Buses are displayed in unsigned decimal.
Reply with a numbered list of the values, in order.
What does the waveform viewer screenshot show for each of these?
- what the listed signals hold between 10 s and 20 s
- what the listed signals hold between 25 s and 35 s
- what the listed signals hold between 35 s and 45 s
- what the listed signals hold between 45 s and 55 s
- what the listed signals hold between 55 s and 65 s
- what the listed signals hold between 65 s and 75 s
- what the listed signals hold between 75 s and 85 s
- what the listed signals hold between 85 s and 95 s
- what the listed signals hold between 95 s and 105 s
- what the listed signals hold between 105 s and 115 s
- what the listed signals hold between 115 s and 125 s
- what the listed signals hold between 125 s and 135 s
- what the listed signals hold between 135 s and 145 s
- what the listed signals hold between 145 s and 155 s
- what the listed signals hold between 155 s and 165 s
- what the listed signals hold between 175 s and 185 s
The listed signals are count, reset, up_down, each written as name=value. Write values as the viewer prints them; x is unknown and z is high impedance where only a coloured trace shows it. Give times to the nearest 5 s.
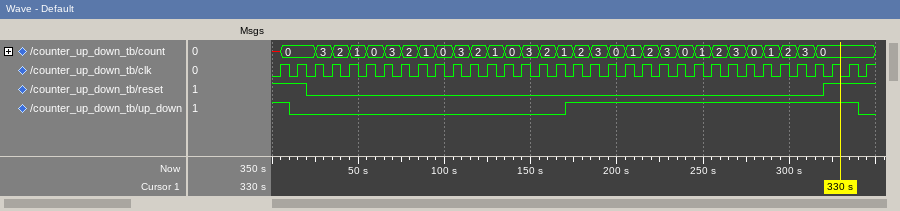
1. count=0, reset=1, up_down=0
2. count=3, reset=0, up_down=0
3. count=2, reset=0, up_down=0
4. count=1, reset=0, up_down=0
5. count=0, reset=0, up_down=0
6. count=3, reset=0, up_down=0
7. count=2, reset=0, up_down=0
8. count=1, reset=0, up_down=0
9. count=0, reset=0, up_down=0
10. count=3, reset=0, up_down=0
11. count=2, reset=0, up_down=0
12. count=1, reset=0, up_down=0
13. count=0, reset=0, up_down=0
14. count=3, reset=0, up_down=0
15. count=2, reset=0, up_down=0
16. count=2, reset=0, up_down=1
